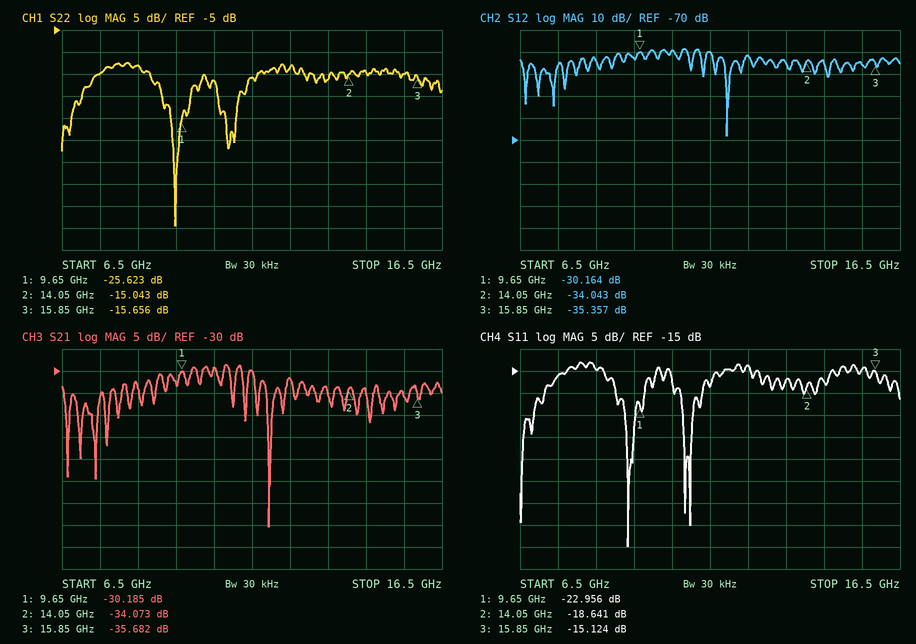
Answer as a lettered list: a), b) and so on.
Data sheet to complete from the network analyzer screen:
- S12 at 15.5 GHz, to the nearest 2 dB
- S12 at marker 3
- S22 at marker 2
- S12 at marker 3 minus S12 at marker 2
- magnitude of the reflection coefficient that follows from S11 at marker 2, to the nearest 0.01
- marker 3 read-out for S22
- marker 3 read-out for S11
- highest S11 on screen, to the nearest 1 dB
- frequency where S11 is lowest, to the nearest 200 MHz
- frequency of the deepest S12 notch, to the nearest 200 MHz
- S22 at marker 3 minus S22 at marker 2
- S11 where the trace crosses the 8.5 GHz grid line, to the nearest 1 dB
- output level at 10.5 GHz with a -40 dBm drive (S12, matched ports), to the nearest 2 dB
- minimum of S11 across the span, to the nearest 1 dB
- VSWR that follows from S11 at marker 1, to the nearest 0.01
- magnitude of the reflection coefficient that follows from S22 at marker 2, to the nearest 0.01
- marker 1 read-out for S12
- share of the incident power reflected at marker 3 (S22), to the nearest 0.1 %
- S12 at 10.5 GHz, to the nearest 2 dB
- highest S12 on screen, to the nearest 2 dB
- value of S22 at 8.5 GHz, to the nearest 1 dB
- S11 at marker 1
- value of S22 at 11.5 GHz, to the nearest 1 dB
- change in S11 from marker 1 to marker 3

a) -36 dB
b) -35.357 dB
c) -15.043 dB
d) -1.314 dB
e) 0.12
f) -15.656 dB
g) -15.124 dB
h) -13 dB
i) 9.4 GHz
j) 12.0 GHz
k) -0.613 dB
l) -15 dB
m) -70 dBm
n) -55 dB
o) 1.15
p) 0.18
q) -30.164 dB
r) 2.7 %
s) -30 dB
t) -28 dB
u) -13 dB
v) -22.956 dB
w) -16 dB
x) 7.832 dB
